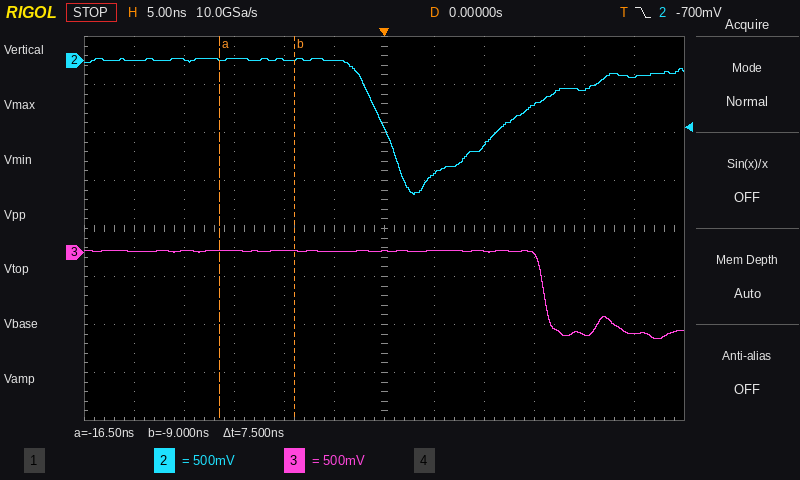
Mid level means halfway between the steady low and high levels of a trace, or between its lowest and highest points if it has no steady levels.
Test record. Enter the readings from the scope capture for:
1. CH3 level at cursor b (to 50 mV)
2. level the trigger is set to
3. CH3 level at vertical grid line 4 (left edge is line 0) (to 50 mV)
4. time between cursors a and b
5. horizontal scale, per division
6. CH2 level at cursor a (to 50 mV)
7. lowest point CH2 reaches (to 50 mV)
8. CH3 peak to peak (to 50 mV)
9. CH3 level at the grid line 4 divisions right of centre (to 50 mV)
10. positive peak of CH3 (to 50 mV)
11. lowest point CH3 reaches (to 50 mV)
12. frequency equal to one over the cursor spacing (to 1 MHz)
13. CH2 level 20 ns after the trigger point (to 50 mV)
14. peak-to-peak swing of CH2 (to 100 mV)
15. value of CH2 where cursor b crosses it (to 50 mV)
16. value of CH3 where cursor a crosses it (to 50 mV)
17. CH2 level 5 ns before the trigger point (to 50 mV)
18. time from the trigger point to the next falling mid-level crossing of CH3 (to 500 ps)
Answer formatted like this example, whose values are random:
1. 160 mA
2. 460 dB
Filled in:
1. 0 mV
2. -700 mV
3. 0 mV
4. 7.5 ns
5. 5 ns
6. 0 mV
7. -1.40 V
8. 900 mV
9. -850 mV
10. 0 mV
11. -900 mV
12. 133 MHz
13. -300 mV
14. 1.40 V
15. 0 mV
16. 0 mV
17. 0 mV
18. 16.0 ns
